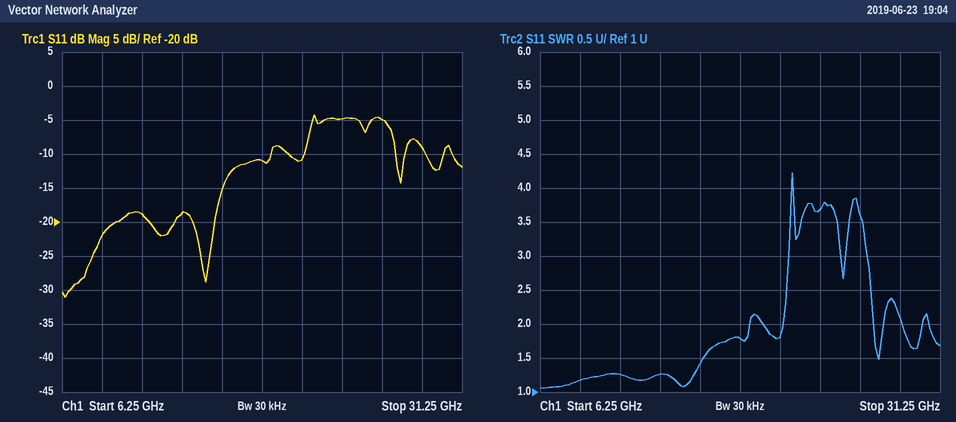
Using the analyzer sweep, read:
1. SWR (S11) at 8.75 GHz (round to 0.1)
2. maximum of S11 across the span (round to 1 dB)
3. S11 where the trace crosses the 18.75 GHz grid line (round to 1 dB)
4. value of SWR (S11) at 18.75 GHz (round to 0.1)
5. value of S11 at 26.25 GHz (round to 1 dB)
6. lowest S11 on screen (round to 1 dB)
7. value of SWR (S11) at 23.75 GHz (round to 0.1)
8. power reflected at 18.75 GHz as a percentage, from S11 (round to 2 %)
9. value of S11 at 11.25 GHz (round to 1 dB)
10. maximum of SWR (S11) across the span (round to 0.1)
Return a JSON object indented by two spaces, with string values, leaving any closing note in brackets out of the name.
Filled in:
{
  "SWR (S11) at 8.75 GHz": "1.2",
  "maximum of S11 across the span": "-4 dB",
  "S11 where the trace crosses the 18.75 GHz grid line": "-11 dB",
  "value of SWR (S11) at 18.75 GHz": "1.8",
  "value of S11 at 26.25 GHz": "-5 dB",
  "lowest S11 on screen": "-31 dB",
  "value of SWR (S11) at 23.75 GHz": "3.7",
  "power reflected at 18.75 GHz as a percentage, from S11": "8 %",
  "value of S11 at 11.25 GHz": "-19 dB",
  "maximum of SWR (S11) across the span": "4.2"
}
